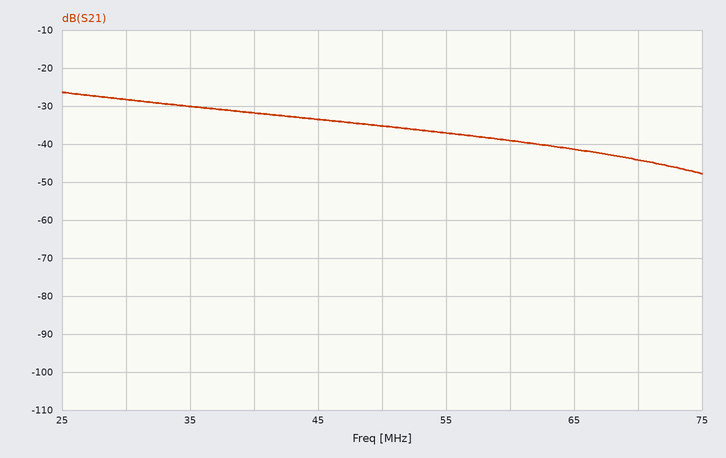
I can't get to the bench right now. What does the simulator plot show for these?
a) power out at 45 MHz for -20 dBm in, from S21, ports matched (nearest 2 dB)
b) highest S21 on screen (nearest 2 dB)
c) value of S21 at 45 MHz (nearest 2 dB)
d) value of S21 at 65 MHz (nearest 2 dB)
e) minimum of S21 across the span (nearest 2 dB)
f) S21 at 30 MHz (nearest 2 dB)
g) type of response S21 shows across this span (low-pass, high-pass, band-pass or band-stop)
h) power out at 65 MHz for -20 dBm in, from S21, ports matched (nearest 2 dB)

-54 dBm
-26 dB
-34 dB
-42 dB
-48 dB
-28 dB
low-pass
-62 dBm
